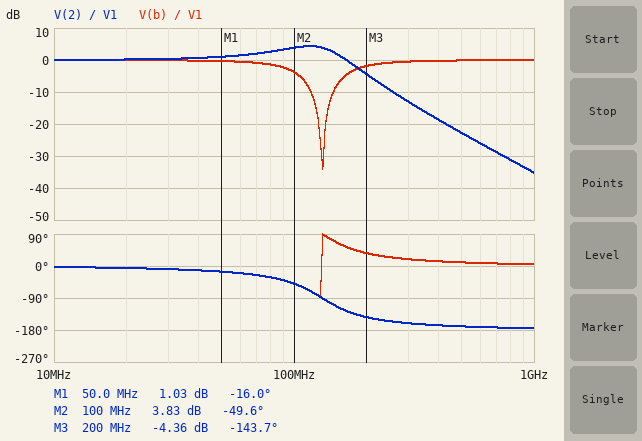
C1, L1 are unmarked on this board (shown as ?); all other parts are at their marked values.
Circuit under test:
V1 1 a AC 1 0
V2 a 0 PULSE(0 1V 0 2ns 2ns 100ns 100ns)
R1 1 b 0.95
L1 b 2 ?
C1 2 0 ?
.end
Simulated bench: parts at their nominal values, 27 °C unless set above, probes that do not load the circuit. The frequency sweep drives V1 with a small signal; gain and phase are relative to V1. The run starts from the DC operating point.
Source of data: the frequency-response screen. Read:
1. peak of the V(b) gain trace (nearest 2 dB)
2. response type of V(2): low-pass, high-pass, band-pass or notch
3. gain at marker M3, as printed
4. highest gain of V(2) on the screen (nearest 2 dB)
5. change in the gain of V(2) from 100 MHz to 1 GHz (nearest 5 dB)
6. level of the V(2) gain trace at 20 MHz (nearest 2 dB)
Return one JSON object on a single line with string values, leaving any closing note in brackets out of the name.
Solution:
{"peak of the V(b) gain trace": "0 dB", "response type of V(2): low-pass, high-pass, band-pass or notch": "low-pass", "gain at marker M3, as printed": "-4.36 dB", "highest gain of V(2) on the screen": "4 dB", "change in the gain of V(2) from 100 MHz to 1 GHz": "-40 dB", "level of the V(2) gain trace at 20 MHz": "0 dB"}
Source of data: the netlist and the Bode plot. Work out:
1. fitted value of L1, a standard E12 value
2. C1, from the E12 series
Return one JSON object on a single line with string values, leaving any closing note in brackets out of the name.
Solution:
{"fitted value of L1, a standard E12 value": "1.8 nH", "C1, from the E12 series": "820 pF"}
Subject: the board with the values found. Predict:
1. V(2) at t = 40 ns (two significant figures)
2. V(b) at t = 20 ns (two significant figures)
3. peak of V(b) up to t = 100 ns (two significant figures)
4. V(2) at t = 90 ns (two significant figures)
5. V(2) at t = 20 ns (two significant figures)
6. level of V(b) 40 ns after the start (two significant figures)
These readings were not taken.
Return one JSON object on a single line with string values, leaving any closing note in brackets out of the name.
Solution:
{"V(2) at t = 40 ns": "1.0 V", "V(b) at t = 20 ns": "1.0 V", "peak of V(b) up to t = 100 ns": "1.1 V", "V(2) at t = 90 ns": "1.0 V", "V(2) at t = 20 ns": "1.0 V", "level of V(b) 40 ns after the start": "1.0 V"}
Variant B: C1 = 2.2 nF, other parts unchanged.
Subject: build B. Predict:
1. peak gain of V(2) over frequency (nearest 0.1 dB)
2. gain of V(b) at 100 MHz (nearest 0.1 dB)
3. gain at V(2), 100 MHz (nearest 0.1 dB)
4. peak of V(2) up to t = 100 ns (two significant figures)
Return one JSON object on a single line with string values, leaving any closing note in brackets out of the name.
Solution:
{"peak gain of V(2) over frequency": "1.0 dB", "gain of V(b) at 100 MHz": "-8.1 dB", "gain at V(2), 100 MHz": "-3.1 dB", "peak of V(2) up to t = 100 ns": "1.1 V"}
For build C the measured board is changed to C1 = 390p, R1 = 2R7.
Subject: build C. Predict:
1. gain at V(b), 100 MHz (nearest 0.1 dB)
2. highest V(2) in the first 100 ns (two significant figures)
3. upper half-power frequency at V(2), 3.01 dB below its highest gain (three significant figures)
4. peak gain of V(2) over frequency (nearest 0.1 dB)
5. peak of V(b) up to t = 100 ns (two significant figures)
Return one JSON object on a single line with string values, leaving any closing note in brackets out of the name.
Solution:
{"gain at V(b), 100 MHz": "-2.6 dB", "highest V(2) in the first 100 ns": "1.1 V", "upper half-power frequency at V(2), 3.01 dB below its highest gain": "207 MHz", "peak gain of V(2) over frequency": "0.2 dB", "peak of V(b) up to t = 100 ns": "1.0 V"}
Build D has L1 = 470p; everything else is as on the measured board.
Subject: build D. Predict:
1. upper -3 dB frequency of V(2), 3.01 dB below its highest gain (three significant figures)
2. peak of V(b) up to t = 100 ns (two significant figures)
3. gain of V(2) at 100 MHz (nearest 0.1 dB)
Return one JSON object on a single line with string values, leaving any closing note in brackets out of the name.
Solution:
{"upper -3 dB frequency of V(2), 3.01 dB below its highest gain": "280 MHz", "peak of V(b) up to t = 100 ns": "1.0 V", "gain of V(2) at 100 MHz": "0.2 dB"}
